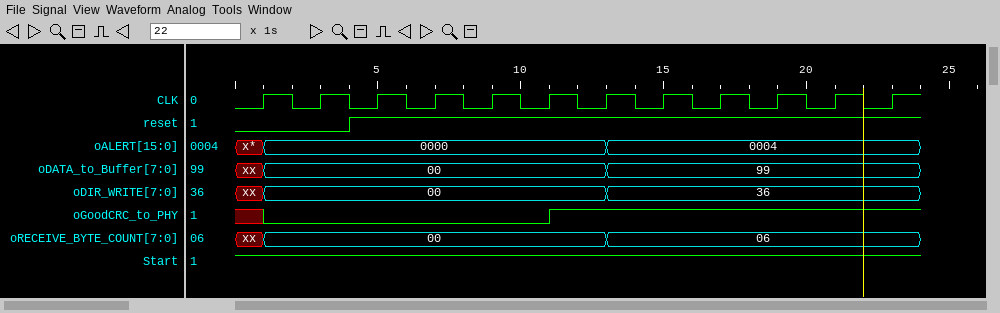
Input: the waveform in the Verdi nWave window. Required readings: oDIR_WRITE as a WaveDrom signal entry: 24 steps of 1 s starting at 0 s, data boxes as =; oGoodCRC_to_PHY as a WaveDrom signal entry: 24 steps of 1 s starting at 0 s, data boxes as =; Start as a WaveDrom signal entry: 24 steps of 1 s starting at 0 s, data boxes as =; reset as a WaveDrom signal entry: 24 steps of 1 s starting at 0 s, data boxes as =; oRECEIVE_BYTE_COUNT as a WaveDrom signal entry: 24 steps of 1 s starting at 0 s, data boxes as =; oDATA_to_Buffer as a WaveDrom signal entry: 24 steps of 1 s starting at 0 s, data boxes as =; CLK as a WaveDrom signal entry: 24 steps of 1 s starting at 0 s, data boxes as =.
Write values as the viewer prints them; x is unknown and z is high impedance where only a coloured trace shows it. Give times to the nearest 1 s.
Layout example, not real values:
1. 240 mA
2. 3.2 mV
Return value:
1. {name: 'oDIR_WRITE', wave: 'x=...........=..........', data: '00 36'}
2. {name: 'oGoodCRC_to_PHY', wave: 'x0.........1............'}
3. {name: 'Start', wave: '1.......................'}
4. {name: 'reset', wave: '0...1...................'}
5. {name: 'oRECEIVE_BYTE_COUNT', wave: 'x=...........=..........', data: '00 06'}
6. {name: 'oDATA_to_Buffer', wave: 'x=...........=..........', data: '00 99'}
7. {name: 'CLK', wave: '010101010101010101010101'}
